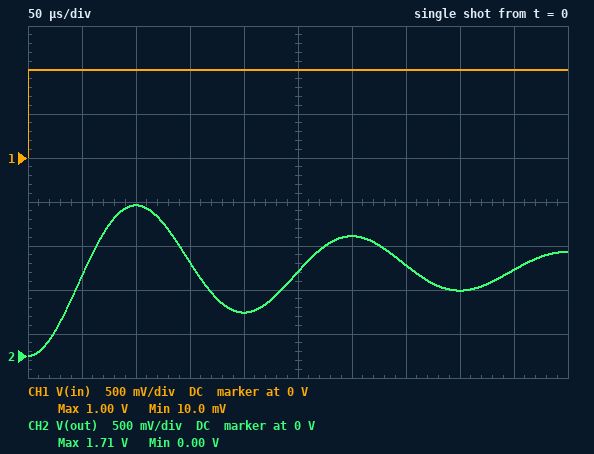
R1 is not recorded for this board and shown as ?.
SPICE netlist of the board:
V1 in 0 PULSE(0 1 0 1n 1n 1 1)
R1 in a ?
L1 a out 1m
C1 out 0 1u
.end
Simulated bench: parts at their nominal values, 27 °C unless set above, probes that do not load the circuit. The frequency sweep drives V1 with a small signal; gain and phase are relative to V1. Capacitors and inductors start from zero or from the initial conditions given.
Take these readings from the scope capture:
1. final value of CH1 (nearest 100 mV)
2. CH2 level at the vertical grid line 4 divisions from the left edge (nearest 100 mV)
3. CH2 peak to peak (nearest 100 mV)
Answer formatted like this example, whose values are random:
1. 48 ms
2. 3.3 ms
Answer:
1. 1.0 V
2. 500 mV
3. 1.7 V
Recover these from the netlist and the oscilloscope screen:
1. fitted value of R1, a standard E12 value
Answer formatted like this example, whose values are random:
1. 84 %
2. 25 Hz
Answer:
1. 6.8 Ω
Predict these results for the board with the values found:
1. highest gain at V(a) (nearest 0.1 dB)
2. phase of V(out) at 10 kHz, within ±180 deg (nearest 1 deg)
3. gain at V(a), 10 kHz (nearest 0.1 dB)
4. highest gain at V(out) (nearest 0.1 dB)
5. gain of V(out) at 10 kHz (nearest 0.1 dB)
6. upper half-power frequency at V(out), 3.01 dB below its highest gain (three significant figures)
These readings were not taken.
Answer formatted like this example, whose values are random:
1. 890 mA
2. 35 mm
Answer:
1. 0 dB
2. -172 deg
3. -0.1 dB
4. 13.4 dB
5. -9.5 dB
6. 5.49 kHz
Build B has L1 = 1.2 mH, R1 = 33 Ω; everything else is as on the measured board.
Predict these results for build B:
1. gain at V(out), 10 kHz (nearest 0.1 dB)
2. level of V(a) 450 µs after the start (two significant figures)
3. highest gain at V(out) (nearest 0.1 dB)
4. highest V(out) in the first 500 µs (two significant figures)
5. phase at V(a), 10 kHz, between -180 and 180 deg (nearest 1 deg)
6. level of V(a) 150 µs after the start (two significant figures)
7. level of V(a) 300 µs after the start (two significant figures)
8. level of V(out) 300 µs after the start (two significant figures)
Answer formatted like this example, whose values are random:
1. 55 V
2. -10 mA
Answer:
1. -12.6 dB
2. 1.0 V
3. 1.5 dB
4. 1.2 V
5. 29 deg
6. 1.1 V
7. 980 mV
8. 990 mV
